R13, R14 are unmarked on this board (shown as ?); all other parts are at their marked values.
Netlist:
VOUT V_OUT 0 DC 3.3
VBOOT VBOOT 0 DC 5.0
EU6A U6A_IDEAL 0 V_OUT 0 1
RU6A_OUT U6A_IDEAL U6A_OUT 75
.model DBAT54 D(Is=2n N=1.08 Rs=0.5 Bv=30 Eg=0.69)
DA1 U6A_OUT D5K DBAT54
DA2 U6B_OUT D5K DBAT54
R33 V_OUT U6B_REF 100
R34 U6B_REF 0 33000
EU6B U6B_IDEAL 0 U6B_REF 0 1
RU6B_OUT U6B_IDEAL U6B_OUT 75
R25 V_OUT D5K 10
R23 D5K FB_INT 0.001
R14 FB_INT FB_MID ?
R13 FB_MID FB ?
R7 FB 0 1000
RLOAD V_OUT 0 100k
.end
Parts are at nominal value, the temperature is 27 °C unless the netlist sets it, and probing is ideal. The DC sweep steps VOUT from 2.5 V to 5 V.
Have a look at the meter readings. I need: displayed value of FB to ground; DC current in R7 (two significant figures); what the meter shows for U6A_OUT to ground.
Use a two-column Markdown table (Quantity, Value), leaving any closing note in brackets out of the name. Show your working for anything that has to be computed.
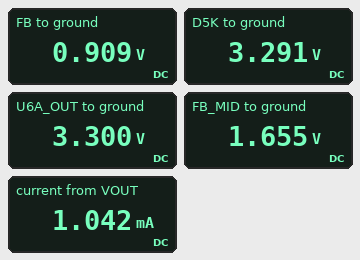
| Quantity | Value |
|---|---|
| displayed value of FB to ground | 0.909 V |
| DC current in R7 | (909 mV) / 1 kΩ = 910 µA |
| what the meter shows for U6A_OUT to ground | 3.300 V |
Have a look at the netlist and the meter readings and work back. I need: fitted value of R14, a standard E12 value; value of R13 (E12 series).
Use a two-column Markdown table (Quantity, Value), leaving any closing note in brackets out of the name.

| Quantity | Value |
|---|---|
| fitted value of R14, a standard E12 value | 1.8 kΩ |
| value of R13 | 820 Ω |
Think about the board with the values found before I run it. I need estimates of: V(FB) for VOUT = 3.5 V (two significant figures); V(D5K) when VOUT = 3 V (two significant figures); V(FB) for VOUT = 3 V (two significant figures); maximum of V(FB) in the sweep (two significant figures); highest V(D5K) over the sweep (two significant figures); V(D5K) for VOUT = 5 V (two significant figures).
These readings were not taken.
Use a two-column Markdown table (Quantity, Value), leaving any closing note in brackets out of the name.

| Quantity | Value |
|---|---|
| V(FB) for VOUT = 3.5 V | 960 mV |
| V(D5K) when VOUT = 3 V | 3.0 V |
| V(FB) for VOUT = 3 V | 830 mV |
| maximum of V(FB) in the sweep | 1.4 V |
| highest V(D5K) over the sweep | 5.0 V |
| V(D5K) for VOUT = 5 V | 5.0 V |
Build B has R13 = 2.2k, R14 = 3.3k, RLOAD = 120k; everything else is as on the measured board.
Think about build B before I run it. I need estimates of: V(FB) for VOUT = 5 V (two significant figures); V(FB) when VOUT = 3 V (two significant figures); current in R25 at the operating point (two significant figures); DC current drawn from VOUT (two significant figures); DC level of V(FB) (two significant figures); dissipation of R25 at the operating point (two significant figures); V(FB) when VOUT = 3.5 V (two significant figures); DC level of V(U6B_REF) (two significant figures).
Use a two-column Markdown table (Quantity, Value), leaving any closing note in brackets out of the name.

| Quantity | Value |
|---|---|
| V(FB) for VOUT = 5 V | 770 mV |
| V(FB) when VOUT = 3 V | 460 mV |
| current in R25 at the operating point | 510 µA |
| DC current drawn from VOUT | 630 µA |
| DC level of V(FB) | 510 mV |
| dissipation of R25 at the operating point | 2.6 µW |
| V(FB) when VOUT = 3.5 V | 540 mV |
| DC level of V(U6B_REF) | 3.3 V |
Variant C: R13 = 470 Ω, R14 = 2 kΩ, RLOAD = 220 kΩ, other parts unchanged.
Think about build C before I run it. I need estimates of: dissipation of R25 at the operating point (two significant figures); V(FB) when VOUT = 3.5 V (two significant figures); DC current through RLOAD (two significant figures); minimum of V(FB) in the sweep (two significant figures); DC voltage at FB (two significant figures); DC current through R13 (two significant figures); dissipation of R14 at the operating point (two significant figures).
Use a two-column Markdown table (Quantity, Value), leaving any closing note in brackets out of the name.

| Quantity | Value |
|---|---|
| dissipation of R25 at the operating point | 9.0 µW |
| V(FB) when VOUT = 3.5 V | 1.0 V |
| DC current through RLOAD | 15 µA |
| minimum of V(FB) in the sweep | 720 mV |
| DC voltage at FB | 950 mV |
| DC current through R13 | 950 µA |
| dissipation of R14 at the operating point | 1.8 mW |
